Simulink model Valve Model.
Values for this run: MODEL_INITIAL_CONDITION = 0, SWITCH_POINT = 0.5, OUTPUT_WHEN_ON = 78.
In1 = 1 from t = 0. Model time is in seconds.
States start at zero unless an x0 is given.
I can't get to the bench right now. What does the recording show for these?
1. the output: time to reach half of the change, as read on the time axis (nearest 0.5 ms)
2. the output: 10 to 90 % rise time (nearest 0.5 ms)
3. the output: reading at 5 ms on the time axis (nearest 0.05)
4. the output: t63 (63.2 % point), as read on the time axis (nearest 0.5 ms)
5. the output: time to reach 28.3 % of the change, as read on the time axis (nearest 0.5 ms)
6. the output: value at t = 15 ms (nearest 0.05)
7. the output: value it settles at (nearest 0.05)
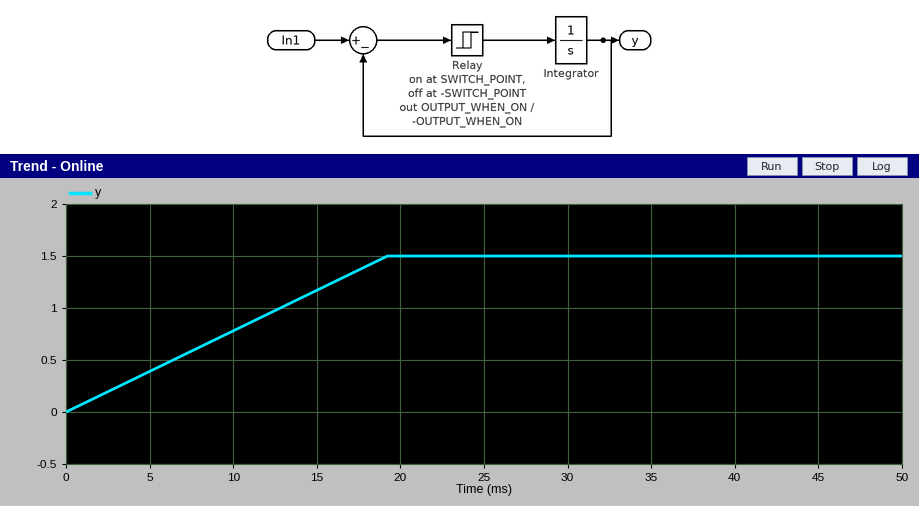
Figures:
9.5 ms
15.5 ms
0.40
12.0 ms
5.5 ms
1.15
1.50
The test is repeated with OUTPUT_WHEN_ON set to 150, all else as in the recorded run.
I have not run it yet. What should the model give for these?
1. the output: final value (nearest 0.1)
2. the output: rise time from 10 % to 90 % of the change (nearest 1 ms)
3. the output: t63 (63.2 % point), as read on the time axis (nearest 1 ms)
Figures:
1.5
8 ms
6 ms
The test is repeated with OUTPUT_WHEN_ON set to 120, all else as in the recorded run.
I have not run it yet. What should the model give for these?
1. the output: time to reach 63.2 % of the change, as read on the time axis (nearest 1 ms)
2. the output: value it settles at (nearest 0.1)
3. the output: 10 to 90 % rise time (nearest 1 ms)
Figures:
8 ms
1.5
10 ms
